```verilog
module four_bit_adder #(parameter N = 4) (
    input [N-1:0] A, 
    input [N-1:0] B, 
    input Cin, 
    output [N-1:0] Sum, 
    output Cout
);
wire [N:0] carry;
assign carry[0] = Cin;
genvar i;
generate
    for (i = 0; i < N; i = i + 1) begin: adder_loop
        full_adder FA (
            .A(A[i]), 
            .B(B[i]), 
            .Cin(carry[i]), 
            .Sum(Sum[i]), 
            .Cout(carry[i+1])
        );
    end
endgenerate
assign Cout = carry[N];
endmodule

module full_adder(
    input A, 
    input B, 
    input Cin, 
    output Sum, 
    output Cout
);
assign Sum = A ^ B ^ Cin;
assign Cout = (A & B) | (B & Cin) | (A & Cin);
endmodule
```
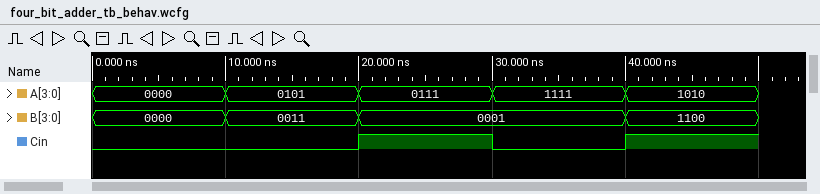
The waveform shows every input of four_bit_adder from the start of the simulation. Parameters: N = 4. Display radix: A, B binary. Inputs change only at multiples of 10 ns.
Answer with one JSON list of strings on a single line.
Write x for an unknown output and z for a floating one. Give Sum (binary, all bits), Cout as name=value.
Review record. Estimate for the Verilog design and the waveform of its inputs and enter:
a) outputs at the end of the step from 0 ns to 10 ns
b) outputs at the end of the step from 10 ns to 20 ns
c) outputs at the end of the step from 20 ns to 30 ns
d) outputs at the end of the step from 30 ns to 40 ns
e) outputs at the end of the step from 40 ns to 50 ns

["Sum=0000, Cout=0", "Sum=1000, Cout=0", "Sum=1001, Cout=0", "Sum=0000, Cout=1", "Sum=0111, Cout=1"]
